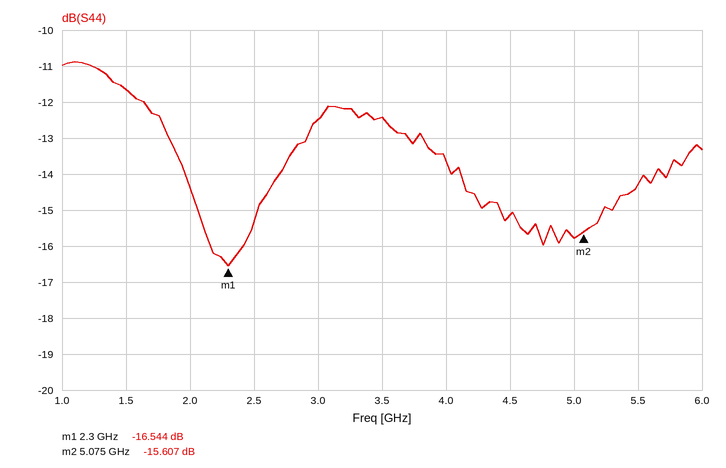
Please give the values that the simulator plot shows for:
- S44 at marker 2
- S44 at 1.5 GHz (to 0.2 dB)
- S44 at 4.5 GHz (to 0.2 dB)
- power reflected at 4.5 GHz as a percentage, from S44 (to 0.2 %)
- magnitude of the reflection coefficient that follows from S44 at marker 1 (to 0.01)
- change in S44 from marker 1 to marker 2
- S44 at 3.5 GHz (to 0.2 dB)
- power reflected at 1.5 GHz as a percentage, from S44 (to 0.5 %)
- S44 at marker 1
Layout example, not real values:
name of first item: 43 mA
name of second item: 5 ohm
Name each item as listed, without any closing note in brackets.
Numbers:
S44 at marker 2: -15.607 dB
S44 at 1.5 GHz: -11.6 dB
S44 at 4.5 GHz: -15.2 dB
power reflected at 4.5 GHz as a percentage, from S44: 3.0 %
magnitude of the reflection coefficient that follows from S44 at marker 1: 0.15
change in S44 from marker 1 to marker 2: 0.937 dB
S44 at 3.5 GHz: -12.4 dB
power reflected at 1.5 GHz as a percentage, from S44: 7.0 %
S44 at marker 1: -16.544 dB
